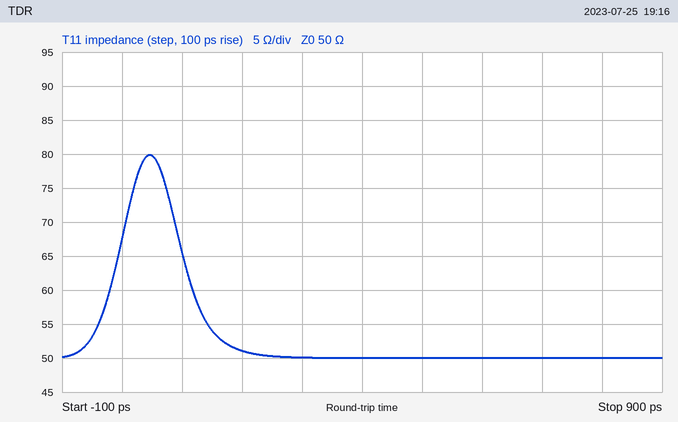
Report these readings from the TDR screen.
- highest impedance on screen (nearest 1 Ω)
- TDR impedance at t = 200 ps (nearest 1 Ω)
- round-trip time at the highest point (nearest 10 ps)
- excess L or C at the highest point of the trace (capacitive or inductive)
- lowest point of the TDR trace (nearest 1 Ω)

80 Ω
51 Ω
50 ps
inductive
50 Ω
